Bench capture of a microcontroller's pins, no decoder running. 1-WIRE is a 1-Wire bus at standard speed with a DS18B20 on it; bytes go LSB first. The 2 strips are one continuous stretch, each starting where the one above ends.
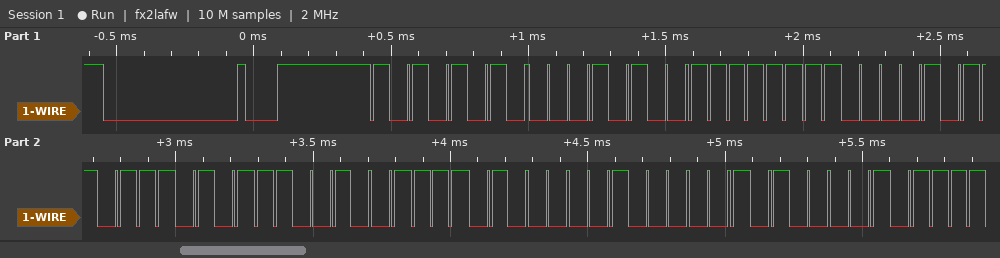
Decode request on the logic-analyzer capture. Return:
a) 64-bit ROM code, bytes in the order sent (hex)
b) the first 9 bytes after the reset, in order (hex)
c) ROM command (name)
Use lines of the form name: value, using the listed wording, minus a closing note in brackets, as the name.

64-bit ROM code, bytes in the order sent: 28 FF D0 AE 93 17 04 85
the first 9 bytes after the reset, in order: 55 28 FF D0 AE 93 17 04 85
ROM command: Match ROM
